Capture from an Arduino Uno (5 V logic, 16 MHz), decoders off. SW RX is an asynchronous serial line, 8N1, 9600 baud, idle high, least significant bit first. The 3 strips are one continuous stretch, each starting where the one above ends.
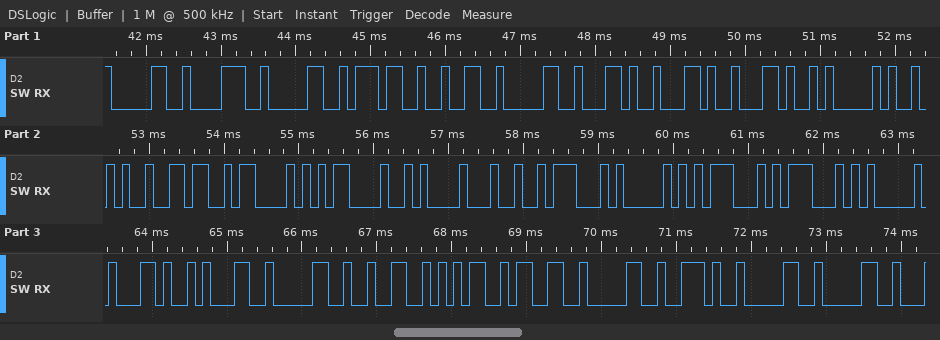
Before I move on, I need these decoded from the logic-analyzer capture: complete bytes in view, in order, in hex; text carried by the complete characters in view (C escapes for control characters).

30 38 30 37 32 30 2C 2C 2C 41 2A 36 43 0D 0A 24 47 50 47 47 41 2C 31 30 32 35 33 30 2E 30 30
"080720,,,A*6C\r\n$GPGGA,102530.00"
